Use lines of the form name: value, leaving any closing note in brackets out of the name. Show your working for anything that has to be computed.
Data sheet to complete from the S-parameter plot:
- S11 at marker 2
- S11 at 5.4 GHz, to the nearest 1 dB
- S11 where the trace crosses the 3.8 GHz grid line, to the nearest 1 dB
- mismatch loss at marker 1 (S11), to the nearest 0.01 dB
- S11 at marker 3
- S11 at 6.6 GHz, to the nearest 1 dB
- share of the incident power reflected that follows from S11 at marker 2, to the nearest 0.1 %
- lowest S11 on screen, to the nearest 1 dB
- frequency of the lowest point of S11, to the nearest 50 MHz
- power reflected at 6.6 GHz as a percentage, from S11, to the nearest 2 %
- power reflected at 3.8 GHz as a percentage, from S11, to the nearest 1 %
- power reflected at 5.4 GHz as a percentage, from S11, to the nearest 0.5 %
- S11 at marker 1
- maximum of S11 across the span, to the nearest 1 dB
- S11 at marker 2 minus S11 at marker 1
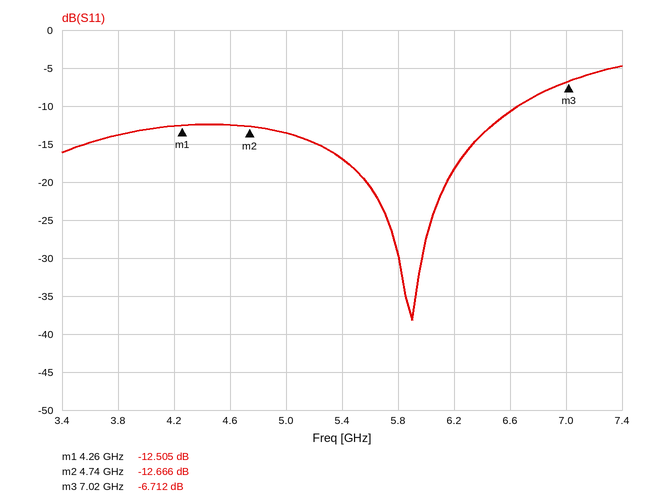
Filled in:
S11 at marker 2: -12.666 dB
S11 at 5.4 GHz, to the nearest 1 dB: -17 dB
S11 where the trace crosses the 3.8 GHz grid line, to the nearest 1 dB: -14 dB
mismatch loss at marker 1 (S11), to the nearest 0.01 dB: −10 log10(1 − 10^(-12.505/10)) ≈ 0.25 dB
S11 at marker 3: -6.712 dB
S11 at 6.6 GHz, to the nearest 1 dB: -11 dB
share of the incident power reflected that follows from S11 at marker 2, to the nearest 0.1 %: 10^(-12.666/10) ≈ 5.4 %
lowest S11 on screen, to the nearest 1 dB: -38 dB
frequency of the lowest point of S11, to the nearest 50 MHz: 5.90 GHz
power reflected at 6.6 GHz as a percentage, from S11, to the nearest 2 %: 10^(-11/10) ≈ 8 %
power reflected at 3.8 GHz as a percentage, from S11, to the nearest 1 %: 10^(-14/10) ≈ 4 %
power reflected at 5.4 GHz as a percentage, from S11, to the nearest 0.5 %: 10^(-17/10) ≈ 2.0 %
S11 at marker 1: -12.505 dB
maximum of S11 across the span, to the nearest 1 dB: -5 dB
S11 at marker 2 minus S11 at marker 1: -12.666 − (-12.505) = -0.161 dB
